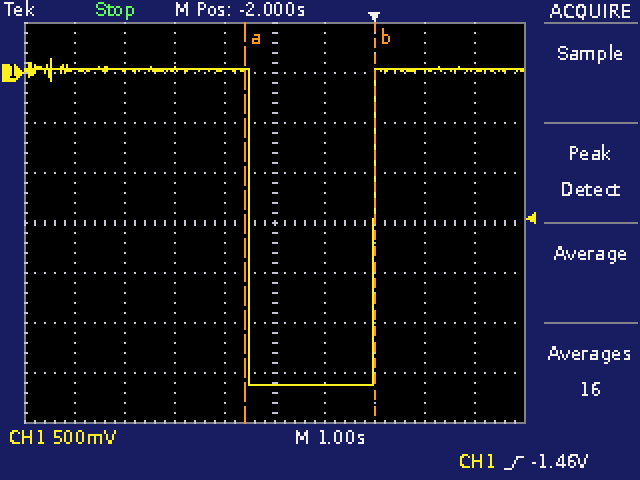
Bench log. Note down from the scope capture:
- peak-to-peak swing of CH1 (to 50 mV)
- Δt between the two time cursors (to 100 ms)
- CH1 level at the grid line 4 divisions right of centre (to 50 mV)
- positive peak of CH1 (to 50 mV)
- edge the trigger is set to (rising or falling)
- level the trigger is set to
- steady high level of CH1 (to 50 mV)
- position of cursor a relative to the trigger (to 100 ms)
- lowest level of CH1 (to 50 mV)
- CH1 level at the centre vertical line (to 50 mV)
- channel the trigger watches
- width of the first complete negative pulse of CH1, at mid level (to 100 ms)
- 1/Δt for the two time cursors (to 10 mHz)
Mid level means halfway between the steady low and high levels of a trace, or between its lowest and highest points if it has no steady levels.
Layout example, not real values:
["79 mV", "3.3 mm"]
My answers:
["3.25 V", "2.6 s", "50 mV", "150 mV", "rising", "-1.46 V", "50 mV", "-2.6 s", "-3.10 V", "-3.10 V", "CH1", "2.5 s", "380 mHz"]
